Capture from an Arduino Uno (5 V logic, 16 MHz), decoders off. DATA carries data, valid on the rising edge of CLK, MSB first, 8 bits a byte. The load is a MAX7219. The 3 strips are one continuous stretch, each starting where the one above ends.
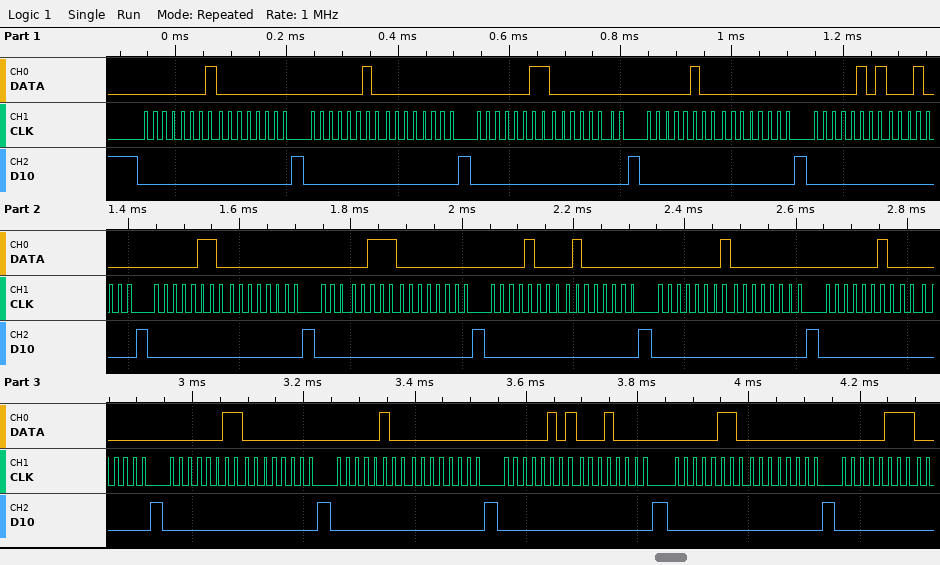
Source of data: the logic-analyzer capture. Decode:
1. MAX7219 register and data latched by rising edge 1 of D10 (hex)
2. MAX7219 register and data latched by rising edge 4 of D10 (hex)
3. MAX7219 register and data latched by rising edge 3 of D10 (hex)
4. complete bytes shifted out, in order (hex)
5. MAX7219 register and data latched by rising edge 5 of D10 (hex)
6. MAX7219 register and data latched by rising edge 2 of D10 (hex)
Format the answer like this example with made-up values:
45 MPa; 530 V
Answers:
register 0x1, data 0x00; register 0x4, data 0x00; register 0x3, data 0x00; 0x01 0x00 0x02 0x00 0x03 0x00 0x04 0x00 0x05 0x10 0x06 0x00 0x07 0x00 0x08 0x40 0x01 0x00 0x02 0x00 0x03 0x00 0x04 0x00 0x05 0x10 0x06 0x00 0x07; register 0x5, data 0x10; register 0x2, data 0x00
